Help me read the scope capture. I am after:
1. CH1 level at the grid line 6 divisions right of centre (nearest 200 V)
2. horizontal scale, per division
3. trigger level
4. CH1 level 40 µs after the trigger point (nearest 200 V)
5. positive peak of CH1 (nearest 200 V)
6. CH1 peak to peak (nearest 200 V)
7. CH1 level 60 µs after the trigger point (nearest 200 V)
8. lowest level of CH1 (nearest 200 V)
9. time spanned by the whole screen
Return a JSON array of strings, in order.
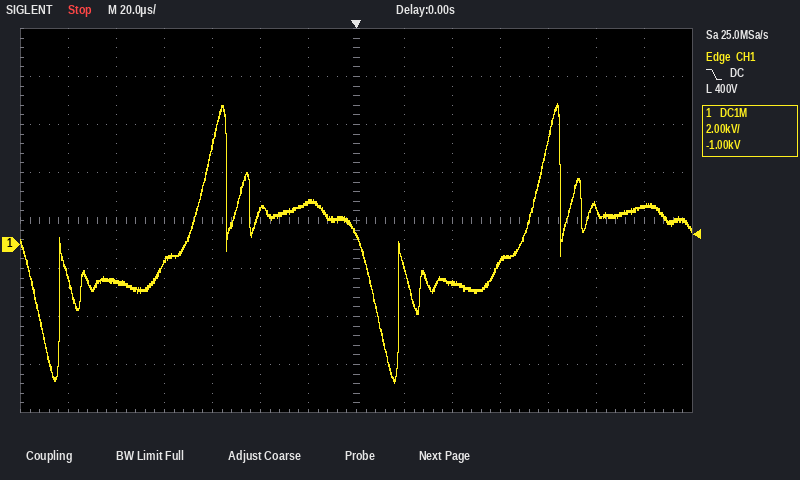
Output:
["1.6 kV", "20 µs", "400 V", "-1.6 kV", "5.8 kV", "11.6 kV", "-800 V", "-5.8 kV", "280 µs"]
